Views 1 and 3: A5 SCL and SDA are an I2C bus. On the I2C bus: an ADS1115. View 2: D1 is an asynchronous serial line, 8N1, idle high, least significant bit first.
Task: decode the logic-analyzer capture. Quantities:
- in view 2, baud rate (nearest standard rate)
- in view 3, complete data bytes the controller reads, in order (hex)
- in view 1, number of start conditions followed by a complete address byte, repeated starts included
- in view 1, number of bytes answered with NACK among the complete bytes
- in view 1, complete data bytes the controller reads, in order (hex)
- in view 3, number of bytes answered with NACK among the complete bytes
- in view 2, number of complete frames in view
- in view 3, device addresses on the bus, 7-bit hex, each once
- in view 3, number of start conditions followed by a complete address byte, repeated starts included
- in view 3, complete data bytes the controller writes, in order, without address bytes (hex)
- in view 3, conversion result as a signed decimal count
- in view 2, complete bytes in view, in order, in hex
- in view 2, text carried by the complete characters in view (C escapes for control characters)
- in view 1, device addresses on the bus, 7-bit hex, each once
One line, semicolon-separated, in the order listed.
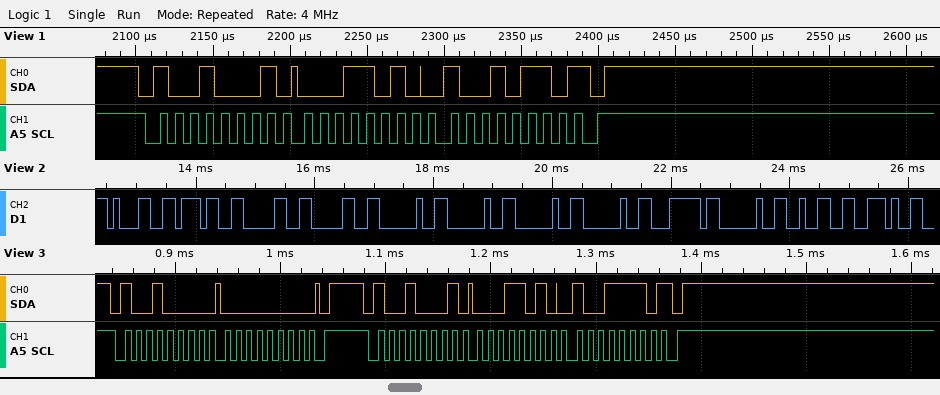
9600 baud; 1A 9E; 1; 1; 1A 96; 1; 12; 0x48; 2; 00; 6814; 31 37 30 30 20 20 20 20 7C 20 32 2E; "1700    | 2."; 0x48
